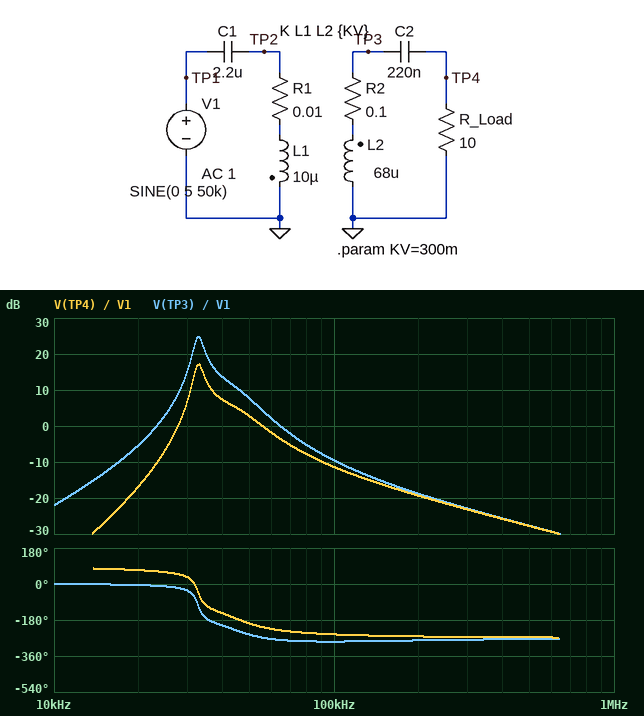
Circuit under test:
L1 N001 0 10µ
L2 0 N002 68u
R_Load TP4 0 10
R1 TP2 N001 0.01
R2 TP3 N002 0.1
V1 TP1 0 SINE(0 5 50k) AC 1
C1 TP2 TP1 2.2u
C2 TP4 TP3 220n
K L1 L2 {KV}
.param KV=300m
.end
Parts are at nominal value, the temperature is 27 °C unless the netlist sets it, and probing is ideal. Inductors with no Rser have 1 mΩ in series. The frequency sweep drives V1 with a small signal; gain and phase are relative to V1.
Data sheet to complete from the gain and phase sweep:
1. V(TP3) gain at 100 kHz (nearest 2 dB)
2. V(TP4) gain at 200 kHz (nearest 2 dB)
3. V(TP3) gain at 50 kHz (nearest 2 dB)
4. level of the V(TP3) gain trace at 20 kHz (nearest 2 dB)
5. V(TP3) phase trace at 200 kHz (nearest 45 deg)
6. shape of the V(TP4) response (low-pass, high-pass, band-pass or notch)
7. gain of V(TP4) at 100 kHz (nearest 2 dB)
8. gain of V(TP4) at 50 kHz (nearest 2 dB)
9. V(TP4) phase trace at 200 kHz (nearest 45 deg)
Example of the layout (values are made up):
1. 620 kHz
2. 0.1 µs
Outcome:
1. -10 dB
2. -20 dB
3. 8 dB
4. -6 dB
5. -270 deg
6. band-pass
7. -12 dB
8. 2 dB
9. -270 deg
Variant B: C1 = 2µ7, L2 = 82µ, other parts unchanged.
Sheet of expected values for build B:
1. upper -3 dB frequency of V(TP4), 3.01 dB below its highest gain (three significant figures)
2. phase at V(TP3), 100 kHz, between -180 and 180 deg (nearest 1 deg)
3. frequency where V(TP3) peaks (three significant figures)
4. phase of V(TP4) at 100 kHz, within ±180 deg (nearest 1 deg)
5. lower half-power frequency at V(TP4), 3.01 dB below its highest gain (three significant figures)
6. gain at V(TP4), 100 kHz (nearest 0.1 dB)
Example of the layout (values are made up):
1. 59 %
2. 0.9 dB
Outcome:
1. 30.8 kHz
2. 69 deg
3. 29.5 kHz
4. 105 deg
5. 28.6 kHz
6. -12.6 dB
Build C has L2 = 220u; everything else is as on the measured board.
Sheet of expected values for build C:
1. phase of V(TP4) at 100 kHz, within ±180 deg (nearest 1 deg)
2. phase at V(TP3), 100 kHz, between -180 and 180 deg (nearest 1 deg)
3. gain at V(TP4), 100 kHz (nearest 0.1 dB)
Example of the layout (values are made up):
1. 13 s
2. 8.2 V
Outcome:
1. 95 deg
2. 59 deg
3. -17.4 dB
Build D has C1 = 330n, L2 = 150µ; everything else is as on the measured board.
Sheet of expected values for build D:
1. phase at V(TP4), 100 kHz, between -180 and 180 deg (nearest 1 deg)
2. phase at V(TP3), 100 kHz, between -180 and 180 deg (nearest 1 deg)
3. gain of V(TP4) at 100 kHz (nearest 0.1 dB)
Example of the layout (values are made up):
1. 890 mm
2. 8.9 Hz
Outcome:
1. 102 deg
2. 66 deg
3. -0.3 dB
